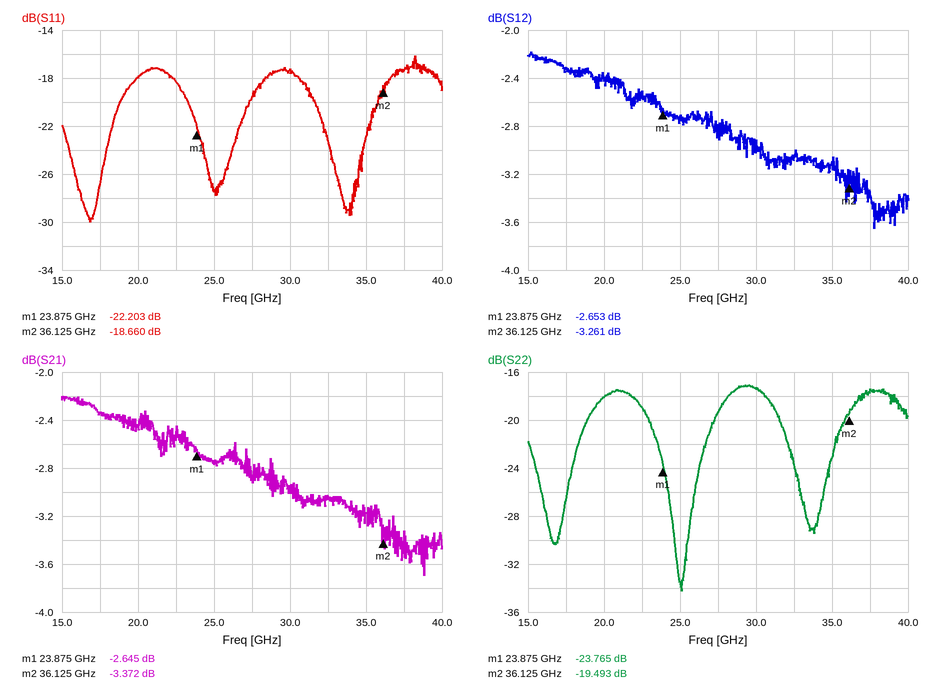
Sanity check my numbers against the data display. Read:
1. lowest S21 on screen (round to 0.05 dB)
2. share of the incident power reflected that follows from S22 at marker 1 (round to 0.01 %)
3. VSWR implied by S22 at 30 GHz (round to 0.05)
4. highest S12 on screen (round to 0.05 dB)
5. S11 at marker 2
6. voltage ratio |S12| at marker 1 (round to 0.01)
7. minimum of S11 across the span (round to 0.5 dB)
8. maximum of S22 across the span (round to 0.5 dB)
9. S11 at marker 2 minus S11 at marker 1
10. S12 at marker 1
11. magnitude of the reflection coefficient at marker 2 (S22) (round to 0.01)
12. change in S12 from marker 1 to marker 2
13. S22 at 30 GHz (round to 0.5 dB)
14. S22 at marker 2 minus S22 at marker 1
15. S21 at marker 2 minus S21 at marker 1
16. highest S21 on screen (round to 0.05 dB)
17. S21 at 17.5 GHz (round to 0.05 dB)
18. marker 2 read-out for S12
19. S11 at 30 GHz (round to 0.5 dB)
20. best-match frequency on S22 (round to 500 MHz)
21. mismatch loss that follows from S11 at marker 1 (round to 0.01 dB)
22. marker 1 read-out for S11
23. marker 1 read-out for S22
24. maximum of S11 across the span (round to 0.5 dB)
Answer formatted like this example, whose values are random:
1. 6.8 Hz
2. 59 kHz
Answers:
1. -3.70 dB
2. 0.42 %
3. 1.30
4. -2.20 dB
5. -18.660 dB
6. 0.74
7. -30.0 dB
8. -17.0 dB
9. 3.543 dB
10. -2.653 dB
11. 0.11
12. -0.608 dB
13. -17.5 dB
14. 4.272 dB
15. -0.727 dB
16. -2.20 dB
17. -2.35 dB
18. -3.261 dB
19. -17.5 dB
20. 25.0 GHz
21. 0.03 dB
22. -22.203 dB
23. -23.765 dB
24. -16.0 dB
